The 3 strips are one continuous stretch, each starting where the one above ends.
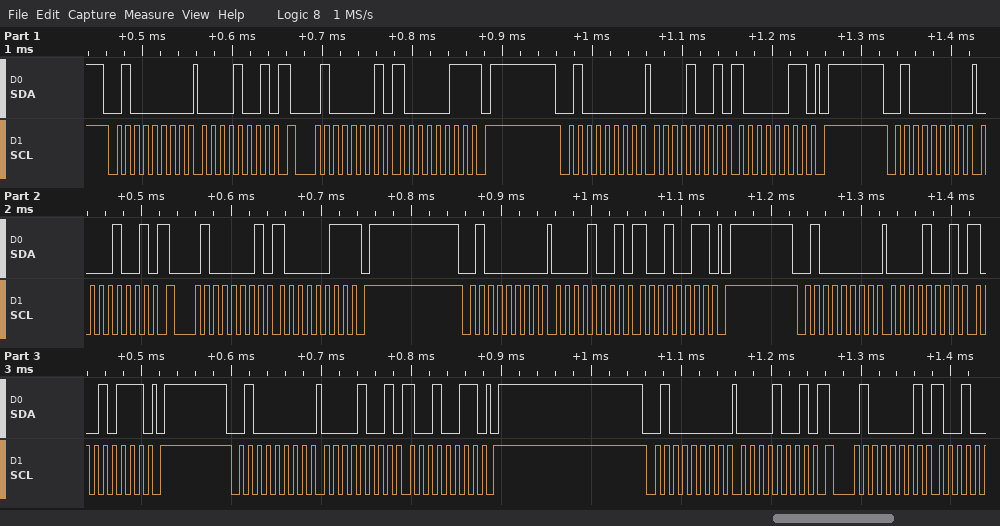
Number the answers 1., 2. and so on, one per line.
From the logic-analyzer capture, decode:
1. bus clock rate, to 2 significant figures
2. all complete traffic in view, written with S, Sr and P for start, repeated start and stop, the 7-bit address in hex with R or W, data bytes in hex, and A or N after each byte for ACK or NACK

1. 100 kHz
2. S 20W A 09 A Sr 20R A 83 N P S 20W A 09 A 83 A P S 20W A 09 A Sr 20R A 83 N P S 20W A 09 A 93 A P S 20W A 09 A 97 A P S 20W A 09 A 93 A P S 20W A 09 A Sr 20R A
